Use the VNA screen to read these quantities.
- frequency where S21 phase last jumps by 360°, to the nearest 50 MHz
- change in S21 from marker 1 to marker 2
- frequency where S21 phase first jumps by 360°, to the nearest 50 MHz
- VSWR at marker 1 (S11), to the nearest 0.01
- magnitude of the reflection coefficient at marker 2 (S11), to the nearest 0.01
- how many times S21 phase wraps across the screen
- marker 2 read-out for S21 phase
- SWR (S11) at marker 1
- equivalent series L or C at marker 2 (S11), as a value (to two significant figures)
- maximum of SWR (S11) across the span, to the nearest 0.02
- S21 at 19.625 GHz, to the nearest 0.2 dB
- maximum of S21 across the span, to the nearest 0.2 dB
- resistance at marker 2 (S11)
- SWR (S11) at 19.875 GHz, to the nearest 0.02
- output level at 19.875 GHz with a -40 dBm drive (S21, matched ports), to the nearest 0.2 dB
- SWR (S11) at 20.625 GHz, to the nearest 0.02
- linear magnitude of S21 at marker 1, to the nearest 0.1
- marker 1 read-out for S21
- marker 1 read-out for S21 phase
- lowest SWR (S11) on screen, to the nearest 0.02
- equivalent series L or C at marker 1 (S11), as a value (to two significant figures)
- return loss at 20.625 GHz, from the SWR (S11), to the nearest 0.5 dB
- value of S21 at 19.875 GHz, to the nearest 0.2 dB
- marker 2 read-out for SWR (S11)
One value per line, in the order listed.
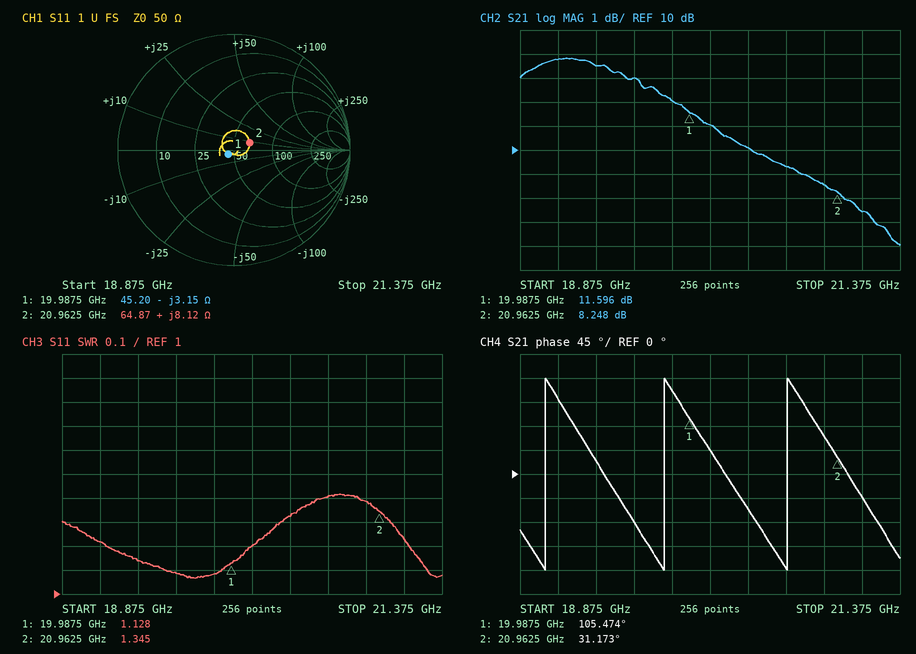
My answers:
20.65 GHz
-3.348 dB
19.05 GHz
1.13
0.15
3
31.173°
1.128
62 pH
1.42
13.0 dB
13.8 dB
64.87 Ω
1.08
-28.0 dBm
1.40
3.8
11.596 dB
105.474°
1.06
2.5 pF
15.5 dB
12.0 dB
1.345
